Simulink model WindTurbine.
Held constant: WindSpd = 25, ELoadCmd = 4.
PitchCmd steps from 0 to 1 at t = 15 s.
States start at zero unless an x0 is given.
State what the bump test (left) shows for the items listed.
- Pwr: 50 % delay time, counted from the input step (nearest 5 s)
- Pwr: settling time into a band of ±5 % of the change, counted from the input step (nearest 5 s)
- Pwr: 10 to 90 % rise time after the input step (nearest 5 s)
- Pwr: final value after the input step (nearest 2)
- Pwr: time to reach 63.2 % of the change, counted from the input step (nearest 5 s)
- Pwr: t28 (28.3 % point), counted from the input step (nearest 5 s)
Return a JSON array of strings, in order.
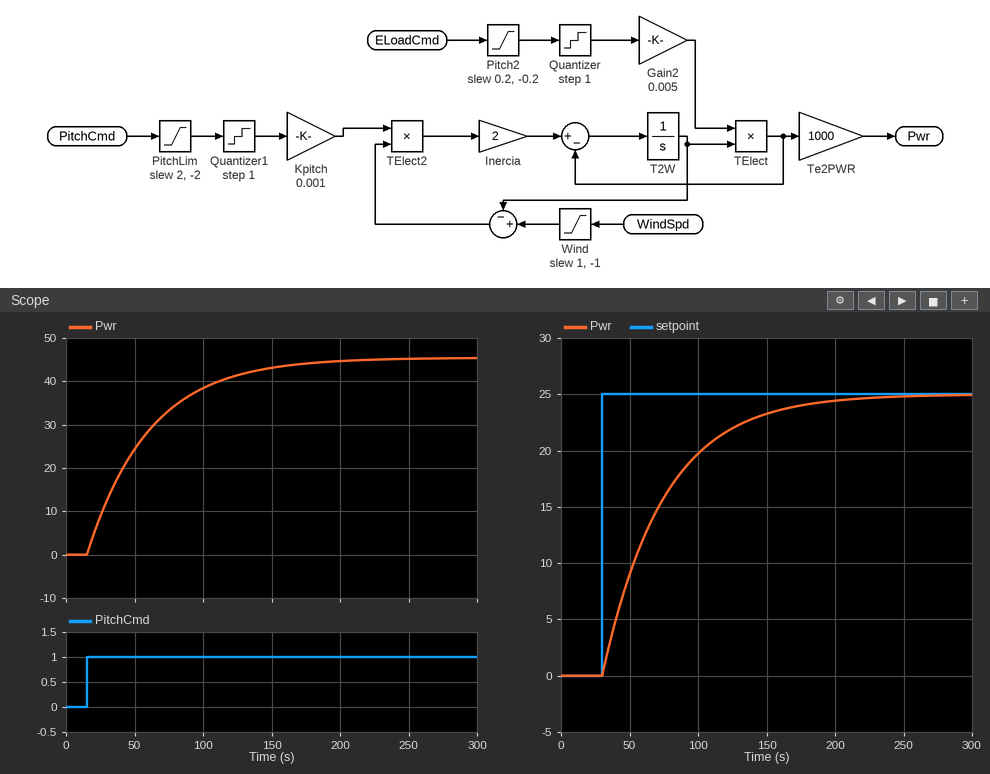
["30 s", "135 s", "100 s", "46", "45 s", "15 s"]
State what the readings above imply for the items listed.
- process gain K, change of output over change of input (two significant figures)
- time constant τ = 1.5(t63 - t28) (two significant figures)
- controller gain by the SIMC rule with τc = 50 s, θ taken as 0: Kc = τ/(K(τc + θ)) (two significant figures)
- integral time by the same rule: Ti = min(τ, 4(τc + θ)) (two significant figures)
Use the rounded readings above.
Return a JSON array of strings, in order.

["46", "45 s", "0.020", "45 s"]
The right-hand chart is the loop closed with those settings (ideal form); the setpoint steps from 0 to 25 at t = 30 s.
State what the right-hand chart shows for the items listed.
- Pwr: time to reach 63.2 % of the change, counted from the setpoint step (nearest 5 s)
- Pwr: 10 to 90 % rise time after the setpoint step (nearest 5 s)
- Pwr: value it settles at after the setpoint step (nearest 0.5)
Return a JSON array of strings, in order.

["45 s", "100 s", "25.0"]
